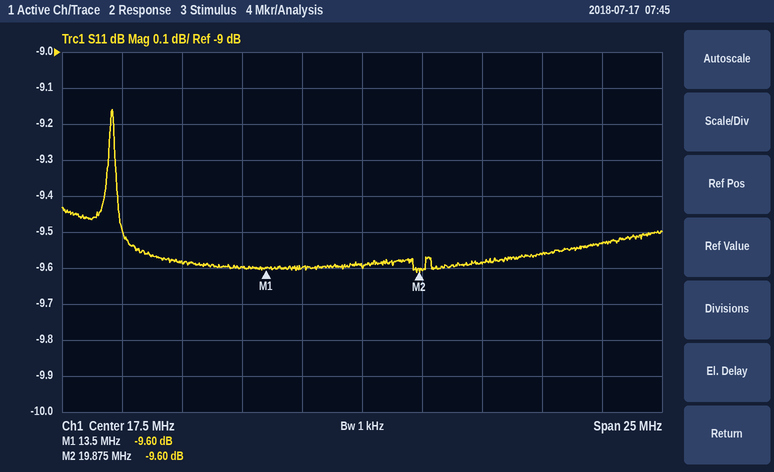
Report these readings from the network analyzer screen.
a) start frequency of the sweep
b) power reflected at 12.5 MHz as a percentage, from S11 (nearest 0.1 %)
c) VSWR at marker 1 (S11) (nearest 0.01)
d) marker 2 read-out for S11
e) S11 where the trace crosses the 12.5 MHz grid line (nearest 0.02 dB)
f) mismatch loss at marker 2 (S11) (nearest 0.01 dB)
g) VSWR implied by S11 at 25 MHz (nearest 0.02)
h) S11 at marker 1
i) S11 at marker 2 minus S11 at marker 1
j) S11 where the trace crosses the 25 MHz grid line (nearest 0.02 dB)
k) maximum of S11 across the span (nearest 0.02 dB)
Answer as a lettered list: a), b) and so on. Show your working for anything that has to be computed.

a) 5 MHz
b) 10^(-9.6/10) ≈ 11.0 %
c) (1 + 0.3311)/(1 − 0.3311) ≈ 1.99
d) -9.60 dB
e) -9.60 dB
f) −10 log10(1 − 10^(-9.6/10)) ≈ 0.50 dB
g) |Γ| = 10^(-9.56/20) = 0.3327; VSWR = (1 + 0.3327)/(1 − 0.3327) ≈ 2.00
h) -9.60 dB
i) -9.6 − (-9.6) = 0.00 dB
j) -9.56 dB
k) -9.16 dB
